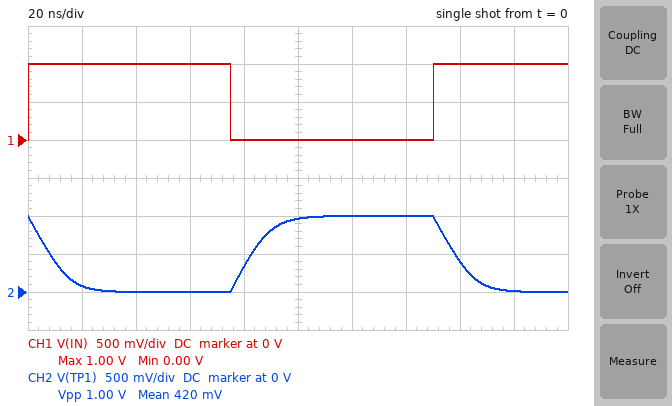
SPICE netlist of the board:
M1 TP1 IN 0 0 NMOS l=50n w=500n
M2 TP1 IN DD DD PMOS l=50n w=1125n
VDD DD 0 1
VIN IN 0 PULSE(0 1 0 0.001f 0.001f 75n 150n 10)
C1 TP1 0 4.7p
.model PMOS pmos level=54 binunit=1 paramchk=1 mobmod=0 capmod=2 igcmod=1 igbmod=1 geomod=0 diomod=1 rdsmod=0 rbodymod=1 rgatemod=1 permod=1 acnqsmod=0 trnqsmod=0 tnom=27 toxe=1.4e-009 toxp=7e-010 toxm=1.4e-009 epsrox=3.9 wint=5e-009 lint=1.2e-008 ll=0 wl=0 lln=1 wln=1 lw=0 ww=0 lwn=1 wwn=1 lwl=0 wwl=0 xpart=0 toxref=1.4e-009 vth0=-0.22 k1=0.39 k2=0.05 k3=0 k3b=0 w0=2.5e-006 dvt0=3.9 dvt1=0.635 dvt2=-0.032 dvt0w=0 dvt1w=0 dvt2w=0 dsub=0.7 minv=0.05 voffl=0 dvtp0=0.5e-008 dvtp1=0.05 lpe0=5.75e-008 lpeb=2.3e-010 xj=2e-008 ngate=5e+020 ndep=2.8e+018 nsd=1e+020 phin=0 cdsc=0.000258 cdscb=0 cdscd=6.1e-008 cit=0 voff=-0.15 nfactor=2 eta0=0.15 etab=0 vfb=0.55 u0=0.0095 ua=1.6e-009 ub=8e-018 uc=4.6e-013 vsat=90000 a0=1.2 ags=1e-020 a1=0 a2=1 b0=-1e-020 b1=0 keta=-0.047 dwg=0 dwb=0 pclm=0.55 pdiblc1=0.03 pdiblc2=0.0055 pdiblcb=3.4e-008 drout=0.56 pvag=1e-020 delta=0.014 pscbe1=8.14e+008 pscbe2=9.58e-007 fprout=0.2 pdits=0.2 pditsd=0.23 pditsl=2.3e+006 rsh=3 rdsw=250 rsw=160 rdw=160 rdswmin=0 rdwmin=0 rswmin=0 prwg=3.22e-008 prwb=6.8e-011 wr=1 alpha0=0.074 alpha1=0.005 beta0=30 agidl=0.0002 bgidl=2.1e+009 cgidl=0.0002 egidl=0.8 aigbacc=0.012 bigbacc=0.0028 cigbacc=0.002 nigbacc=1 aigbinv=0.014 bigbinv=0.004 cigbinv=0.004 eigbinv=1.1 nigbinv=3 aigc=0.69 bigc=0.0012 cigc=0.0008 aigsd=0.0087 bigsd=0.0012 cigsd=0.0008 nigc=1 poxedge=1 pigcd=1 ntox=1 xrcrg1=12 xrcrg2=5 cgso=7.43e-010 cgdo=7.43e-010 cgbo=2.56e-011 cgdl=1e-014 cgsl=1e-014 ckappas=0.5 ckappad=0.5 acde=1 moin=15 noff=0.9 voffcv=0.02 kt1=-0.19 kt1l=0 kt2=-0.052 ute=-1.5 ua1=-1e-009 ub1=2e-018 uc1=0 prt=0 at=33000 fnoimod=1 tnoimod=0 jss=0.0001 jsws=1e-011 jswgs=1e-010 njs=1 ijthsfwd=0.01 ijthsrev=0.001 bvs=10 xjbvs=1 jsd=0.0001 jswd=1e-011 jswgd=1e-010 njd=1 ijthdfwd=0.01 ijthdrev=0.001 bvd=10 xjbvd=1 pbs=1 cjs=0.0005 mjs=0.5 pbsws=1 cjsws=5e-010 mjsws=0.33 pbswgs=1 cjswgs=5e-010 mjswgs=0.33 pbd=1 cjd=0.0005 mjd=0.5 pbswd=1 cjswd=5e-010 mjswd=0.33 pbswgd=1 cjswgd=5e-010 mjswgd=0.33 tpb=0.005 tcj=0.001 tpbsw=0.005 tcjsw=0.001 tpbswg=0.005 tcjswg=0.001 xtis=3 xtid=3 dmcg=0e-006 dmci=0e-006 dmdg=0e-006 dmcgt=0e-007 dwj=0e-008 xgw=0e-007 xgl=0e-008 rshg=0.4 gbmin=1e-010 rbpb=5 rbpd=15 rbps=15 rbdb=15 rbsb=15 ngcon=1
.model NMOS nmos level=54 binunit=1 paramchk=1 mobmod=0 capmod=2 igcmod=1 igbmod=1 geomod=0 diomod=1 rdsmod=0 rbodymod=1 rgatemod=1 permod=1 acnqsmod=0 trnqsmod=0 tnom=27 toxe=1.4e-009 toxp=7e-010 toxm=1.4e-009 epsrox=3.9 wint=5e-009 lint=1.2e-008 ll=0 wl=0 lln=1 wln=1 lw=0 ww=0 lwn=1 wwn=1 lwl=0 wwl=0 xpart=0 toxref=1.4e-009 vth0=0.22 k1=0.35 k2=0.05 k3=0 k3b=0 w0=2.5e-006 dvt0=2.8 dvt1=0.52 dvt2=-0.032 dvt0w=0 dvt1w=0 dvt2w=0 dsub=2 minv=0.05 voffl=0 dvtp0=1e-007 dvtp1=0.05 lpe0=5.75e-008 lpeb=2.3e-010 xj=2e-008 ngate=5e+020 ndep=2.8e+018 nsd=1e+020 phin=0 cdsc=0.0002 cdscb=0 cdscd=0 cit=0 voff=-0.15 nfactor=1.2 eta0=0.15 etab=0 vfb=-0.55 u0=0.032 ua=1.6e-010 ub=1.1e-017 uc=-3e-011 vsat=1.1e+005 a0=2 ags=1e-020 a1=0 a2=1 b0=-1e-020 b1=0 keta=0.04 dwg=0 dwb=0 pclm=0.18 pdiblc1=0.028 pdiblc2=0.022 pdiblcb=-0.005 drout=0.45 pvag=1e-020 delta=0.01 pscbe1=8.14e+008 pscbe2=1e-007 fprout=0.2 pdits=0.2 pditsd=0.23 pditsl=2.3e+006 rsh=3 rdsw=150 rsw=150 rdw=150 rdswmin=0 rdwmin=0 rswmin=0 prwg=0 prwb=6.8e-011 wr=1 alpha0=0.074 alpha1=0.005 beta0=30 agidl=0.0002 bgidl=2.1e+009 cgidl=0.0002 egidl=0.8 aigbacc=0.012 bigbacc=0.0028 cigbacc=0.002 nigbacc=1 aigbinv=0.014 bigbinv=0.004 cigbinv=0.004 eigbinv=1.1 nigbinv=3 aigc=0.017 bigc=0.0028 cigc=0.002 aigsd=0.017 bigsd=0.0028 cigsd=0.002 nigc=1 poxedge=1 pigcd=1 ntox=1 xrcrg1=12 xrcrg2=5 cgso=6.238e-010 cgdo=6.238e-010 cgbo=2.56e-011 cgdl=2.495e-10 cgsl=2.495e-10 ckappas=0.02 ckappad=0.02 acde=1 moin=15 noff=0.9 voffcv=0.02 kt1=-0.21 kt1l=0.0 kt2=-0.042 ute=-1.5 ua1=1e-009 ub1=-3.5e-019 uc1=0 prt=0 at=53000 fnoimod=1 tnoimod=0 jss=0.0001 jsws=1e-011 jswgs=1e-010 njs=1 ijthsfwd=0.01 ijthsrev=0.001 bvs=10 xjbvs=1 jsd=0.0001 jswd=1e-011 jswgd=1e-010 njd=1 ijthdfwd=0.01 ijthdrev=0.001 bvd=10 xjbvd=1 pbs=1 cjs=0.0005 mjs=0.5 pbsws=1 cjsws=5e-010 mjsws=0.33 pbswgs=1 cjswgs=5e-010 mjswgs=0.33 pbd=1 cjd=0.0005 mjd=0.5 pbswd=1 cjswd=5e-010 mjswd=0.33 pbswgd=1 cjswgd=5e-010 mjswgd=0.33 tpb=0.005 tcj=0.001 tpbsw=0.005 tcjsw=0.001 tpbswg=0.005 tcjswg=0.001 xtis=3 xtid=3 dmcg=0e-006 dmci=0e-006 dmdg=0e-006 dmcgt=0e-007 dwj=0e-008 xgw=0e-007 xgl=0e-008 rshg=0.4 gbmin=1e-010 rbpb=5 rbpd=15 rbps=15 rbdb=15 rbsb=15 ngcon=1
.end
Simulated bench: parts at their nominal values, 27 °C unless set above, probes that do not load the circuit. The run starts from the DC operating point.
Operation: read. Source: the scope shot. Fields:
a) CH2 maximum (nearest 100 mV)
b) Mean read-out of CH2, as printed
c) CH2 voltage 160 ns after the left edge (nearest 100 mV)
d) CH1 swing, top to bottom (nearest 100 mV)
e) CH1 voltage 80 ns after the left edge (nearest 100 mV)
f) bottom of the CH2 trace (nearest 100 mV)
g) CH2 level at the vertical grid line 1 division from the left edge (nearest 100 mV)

1.0 V
420 mV
400 mV
1.0 V
0 V
0 V
100 mV
